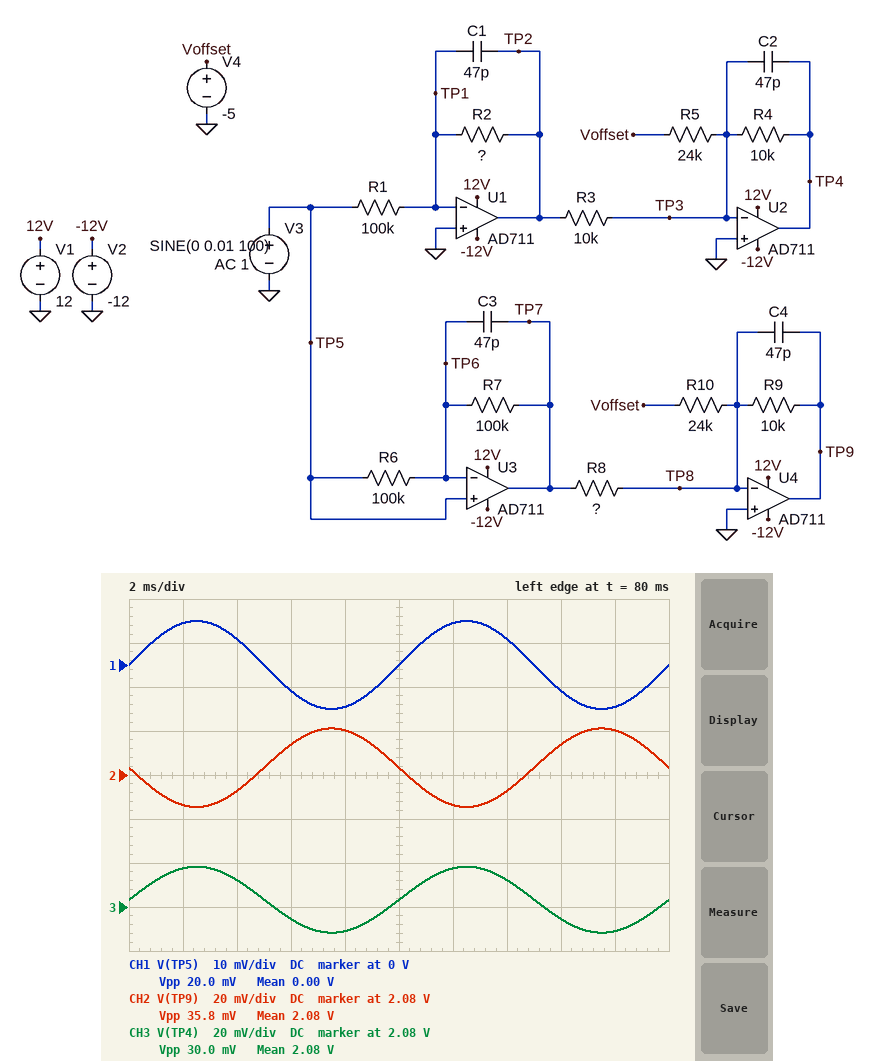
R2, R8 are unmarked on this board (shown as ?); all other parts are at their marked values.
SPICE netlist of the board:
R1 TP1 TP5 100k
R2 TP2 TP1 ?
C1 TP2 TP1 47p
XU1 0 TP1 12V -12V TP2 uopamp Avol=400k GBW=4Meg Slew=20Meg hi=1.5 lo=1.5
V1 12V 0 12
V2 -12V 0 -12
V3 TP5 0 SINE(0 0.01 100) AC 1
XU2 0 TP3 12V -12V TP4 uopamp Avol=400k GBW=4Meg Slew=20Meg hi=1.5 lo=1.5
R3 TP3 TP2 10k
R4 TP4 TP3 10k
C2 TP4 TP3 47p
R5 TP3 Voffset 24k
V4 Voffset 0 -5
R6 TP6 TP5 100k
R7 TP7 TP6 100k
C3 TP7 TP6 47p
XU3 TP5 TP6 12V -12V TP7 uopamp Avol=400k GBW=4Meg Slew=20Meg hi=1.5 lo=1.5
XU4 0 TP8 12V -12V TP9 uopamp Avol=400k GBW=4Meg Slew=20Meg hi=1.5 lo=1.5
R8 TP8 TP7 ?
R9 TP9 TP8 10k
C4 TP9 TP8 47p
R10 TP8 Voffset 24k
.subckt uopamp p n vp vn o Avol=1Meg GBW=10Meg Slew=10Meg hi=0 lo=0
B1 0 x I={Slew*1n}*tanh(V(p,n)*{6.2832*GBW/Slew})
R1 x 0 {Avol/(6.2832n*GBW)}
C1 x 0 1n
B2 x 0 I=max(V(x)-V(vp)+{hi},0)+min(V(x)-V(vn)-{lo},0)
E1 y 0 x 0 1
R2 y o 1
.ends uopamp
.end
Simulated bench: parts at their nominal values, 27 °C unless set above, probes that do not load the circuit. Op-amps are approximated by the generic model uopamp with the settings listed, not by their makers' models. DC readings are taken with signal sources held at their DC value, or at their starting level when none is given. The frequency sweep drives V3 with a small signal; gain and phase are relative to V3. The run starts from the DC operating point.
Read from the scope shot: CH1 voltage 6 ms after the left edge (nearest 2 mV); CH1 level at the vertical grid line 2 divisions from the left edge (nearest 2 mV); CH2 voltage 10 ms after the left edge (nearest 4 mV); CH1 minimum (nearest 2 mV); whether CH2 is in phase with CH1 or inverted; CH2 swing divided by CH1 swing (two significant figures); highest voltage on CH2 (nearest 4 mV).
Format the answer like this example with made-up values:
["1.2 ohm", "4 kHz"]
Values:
["-6 mV", "6 mV", "2.084 V", "-10 mV", "inverted", "1.8", "2.100 V"]
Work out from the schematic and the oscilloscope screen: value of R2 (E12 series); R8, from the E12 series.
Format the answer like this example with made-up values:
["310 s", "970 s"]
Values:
["150 kΩ", "5.6 kΩ"]
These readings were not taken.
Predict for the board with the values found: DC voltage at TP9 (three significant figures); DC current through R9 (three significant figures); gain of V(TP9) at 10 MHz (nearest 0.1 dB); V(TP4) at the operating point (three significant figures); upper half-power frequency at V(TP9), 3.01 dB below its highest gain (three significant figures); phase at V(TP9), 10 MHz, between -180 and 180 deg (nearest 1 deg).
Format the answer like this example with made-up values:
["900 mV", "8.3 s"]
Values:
["2.08 V", "208 µA", "-41.8 dB", "2.08 V", "275 kHz", "-41 deg"]
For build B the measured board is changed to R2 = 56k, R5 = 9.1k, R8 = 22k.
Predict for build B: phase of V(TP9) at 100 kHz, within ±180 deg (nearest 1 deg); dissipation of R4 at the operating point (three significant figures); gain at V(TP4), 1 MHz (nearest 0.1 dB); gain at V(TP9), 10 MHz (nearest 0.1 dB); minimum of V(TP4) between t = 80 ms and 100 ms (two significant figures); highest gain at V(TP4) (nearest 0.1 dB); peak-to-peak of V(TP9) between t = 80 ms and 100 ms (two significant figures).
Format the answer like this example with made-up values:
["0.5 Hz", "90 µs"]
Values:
["159 deg", "3.02 mW", "-41.2 dB", "-53.5 dB", "5.5 V", "-5.0 dB", "9.1 mV"]
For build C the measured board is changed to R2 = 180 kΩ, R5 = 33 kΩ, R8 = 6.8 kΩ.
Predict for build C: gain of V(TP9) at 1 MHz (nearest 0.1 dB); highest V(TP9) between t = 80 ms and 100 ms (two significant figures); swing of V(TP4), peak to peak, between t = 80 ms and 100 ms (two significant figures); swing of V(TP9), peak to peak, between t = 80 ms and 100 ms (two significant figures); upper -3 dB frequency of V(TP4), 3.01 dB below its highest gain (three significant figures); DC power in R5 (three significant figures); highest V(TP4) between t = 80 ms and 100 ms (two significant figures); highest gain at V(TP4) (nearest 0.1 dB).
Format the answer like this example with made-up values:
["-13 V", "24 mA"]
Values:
["-8.3 dB", "2.1 V", "36 mV", "29 mV", "18.6 kHz", "758 µW", "1.5 V", "5.1 dB"]
